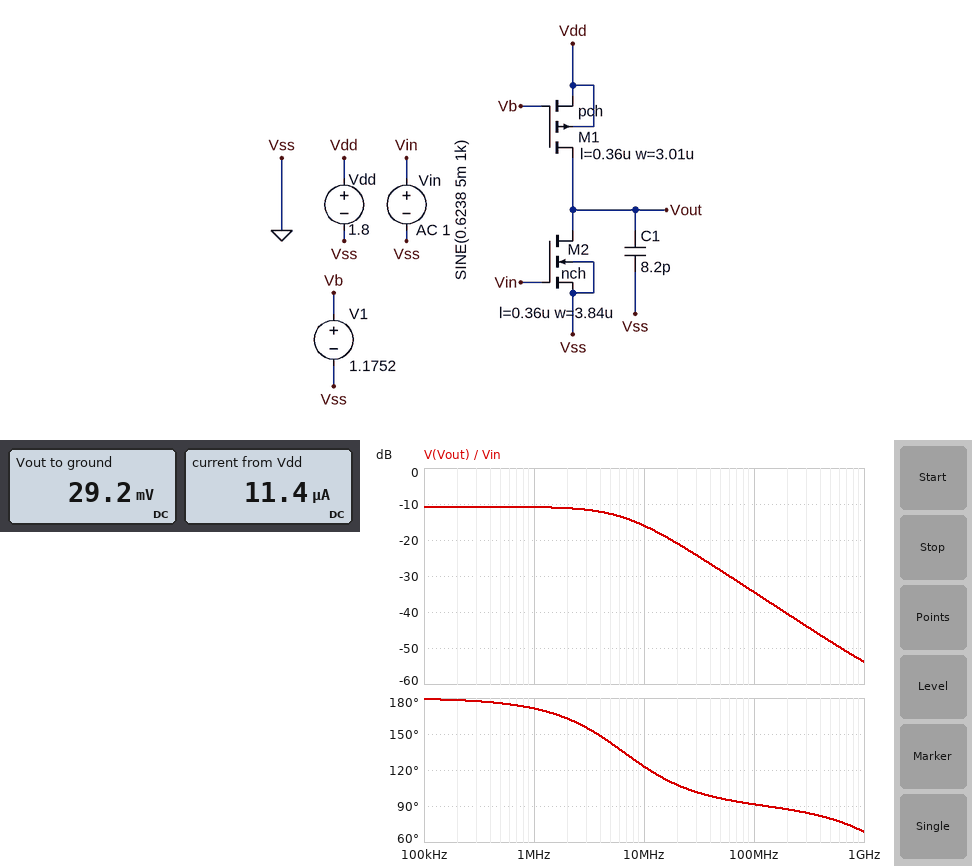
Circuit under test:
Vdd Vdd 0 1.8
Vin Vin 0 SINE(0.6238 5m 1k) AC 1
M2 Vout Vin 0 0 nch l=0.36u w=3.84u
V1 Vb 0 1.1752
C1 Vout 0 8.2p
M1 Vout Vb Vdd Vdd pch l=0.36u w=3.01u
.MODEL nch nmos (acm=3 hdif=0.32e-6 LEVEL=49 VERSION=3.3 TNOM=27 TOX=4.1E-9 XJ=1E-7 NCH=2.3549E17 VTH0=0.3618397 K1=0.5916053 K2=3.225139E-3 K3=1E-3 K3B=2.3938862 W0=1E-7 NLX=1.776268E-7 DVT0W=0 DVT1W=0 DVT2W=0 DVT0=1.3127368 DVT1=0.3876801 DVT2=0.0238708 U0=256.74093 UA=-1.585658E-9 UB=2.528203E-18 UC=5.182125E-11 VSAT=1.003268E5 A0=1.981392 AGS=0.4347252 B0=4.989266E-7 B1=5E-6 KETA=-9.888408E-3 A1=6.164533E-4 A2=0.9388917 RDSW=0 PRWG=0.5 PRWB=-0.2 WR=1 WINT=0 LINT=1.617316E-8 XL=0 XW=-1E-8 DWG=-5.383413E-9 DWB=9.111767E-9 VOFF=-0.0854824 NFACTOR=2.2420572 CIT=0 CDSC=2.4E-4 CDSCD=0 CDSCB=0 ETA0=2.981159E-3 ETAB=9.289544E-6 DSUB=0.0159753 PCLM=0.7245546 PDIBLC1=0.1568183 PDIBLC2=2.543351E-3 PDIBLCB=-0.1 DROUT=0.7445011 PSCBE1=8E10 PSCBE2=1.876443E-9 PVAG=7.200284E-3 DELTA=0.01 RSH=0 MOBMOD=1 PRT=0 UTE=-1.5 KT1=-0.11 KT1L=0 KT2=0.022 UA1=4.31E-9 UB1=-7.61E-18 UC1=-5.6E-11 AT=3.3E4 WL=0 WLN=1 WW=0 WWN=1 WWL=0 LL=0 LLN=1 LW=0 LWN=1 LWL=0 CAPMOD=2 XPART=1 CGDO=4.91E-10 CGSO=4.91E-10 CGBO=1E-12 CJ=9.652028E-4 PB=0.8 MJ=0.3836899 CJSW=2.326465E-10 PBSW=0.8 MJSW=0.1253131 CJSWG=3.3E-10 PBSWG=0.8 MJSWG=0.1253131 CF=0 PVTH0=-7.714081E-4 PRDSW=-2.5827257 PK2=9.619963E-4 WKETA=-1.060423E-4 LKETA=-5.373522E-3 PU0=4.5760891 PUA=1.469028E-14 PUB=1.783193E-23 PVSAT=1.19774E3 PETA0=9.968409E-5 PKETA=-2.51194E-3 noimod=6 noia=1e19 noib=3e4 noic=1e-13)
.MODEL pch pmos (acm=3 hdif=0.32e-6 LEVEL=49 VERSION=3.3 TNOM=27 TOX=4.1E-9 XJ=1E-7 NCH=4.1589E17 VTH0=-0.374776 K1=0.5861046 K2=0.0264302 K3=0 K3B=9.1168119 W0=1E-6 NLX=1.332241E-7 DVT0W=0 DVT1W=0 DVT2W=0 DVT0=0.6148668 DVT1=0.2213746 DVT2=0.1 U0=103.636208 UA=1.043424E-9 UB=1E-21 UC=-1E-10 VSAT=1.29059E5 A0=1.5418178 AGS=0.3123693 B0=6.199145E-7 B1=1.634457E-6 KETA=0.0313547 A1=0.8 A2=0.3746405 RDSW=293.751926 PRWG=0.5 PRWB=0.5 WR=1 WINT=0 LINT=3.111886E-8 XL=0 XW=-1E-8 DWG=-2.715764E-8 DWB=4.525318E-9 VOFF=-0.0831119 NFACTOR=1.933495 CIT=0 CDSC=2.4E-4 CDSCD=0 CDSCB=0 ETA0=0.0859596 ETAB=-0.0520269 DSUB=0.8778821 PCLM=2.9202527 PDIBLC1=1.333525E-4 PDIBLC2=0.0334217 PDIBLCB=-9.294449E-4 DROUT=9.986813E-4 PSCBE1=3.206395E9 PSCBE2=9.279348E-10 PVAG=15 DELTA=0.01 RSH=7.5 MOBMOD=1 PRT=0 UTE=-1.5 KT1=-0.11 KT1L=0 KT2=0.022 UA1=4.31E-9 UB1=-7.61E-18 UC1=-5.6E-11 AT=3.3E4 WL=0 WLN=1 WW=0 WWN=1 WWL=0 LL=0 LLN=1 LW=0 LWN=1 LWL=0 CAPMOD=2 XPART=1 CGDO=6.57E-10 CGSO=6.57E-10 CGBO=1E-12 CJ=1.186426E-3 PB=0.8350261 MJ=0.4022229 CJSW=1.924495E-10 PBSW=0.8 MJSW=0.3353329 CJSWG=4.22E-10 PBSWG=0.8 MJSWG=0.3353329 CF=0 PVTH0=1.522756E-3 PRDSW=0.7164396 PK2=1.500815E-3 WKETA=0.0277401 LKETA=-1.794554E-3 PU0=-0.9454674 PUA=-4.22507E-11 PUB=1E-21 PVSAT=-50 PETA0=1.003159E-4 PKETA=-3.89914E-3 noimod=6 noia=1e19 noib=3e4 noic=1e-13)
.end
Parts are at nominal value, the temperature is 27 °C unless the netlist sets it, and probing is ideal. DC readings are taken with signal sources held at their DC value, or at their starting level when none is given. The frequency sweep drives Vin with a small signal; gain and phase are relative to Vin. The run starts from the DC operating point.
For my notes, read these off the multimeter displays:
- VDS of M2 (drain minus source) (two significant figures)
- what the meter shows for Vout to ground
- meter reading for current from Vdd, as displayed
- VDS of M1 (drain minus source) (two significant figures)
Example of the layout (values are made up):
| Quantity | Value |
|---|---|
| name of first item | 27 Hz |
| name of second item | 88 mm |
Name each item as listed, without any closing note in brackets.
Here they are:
| Quantity | Value |
|---|---|
| VDS of M2 (drain minus source) | 29 mV |
| what the meter shows for Vout to ground | 29.2 mV |
| meter reading for current from Vdd, as displayed | 11.4 µA |
| VDS of M1 (drain minus source) | -1.8 V |
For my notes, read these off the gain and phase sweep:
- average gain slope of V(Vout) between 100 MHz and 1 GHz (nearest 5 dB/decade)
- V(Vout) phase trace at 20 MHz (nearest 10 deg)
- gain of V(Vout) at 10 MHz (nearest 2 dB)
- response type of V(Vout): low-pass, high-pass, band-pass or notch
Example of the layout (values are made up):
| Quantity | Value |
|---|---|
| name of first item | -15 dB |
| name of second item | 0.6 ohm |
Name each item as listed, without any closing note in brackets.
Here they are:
| Quantity | Value |
|---|---|
| average gain slope of V(Vout) between 100 MHz and 1 GHz | -20 dB/decade |
| V(Vout) phase trace at 20 MHz | 110 deg |
| gain of V(Vout) at 10 MHz | -16 dB |
| response type of V(Vout): low-pass, high-pass, band-pass or notch | low-pass |
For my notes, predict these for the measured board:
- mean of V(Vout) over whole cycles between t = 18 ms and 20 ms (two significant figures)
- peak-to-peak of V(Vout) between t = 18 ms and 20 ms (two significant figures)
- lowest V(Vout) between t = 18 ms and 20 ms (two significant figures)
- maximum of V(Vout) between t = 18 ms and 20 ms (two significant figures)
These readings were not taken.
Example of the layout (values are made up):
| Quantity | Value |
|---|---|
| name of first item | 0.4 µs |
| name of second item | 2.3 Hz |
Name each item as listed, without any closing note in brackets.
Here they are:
| Quantity | Value |
|---|---|
| mean of V(Vout) over whole cycles between t = 18 ms and 20 ms | 29 mV |
| peak-to-peak of V(Vout) between t = 18 ms and 20 ms | 2.9 mV |
| lowest V(Vout) between t = 18 ms and 20 ms | 28 mV |
| maximum of V(Vout) between t = 18 ms and 20 ms | 31 mV |
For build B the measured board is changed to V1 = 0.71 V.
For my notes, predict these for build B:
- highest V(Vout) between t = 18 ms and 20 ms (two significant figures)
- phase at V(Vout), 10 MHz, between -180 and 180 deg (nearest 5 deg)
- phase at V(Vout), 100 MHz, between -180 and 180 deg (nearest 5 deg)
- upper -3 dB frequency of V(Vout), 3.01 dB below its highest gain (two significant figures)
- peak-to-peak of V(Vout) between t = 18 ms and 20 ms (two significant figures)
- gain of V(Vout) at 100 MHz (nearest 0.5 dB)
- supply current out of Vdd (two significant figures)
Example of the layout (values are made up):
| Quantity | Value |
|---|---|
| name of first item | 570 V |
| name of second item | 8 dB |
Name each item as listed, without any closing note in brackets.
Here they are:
| Quantity | Value |
|---|---|
| highest V(Vout) between t = 18 ms and 20 ms | 1.7 V |
| phase at V(Vout), 10 MHz, between -180 and 180 deg | 120 deg |
| phase at V(Vout), 100 MHz, between -180 and 180 deg | 95 deg |
| upper -3 dB frequency of V(Vout), 3.01 dB below its highest gain | 5.7 MHz |
| peak-to-peak of V(Vout) between t = 18 ms and 20 ms | 16 mV |
| gain of V(Vout) at 100 MHz | -21.0 dB |
| supply current out of Vdd | 40 µA |
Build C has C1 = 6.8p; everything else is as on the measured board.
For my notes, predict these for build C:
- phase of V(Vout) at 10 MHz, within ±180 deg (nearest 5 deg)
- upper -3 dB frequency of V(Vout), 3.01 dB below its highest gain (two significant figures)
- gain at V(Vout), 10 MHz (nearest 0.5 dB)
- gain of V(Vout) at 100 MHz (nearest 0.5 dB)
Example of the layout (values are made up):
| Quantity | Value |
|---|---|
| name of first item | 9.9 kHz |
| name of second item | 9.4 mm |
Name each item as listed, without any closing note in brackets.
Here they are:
| Quantity | Value |
|---|---|
| phase of V(Vout) at 10 MHz, within ±180 deg | 130 deg |
| upper -3 dB frequency of V(Vout), 3.01 dB below its highest gain | 7.9 MHz |
| gain at V(Vout), 10 MHz | -15.0 dB |
| gain of V(Vout) at 100 MHz | -33.0 dB |
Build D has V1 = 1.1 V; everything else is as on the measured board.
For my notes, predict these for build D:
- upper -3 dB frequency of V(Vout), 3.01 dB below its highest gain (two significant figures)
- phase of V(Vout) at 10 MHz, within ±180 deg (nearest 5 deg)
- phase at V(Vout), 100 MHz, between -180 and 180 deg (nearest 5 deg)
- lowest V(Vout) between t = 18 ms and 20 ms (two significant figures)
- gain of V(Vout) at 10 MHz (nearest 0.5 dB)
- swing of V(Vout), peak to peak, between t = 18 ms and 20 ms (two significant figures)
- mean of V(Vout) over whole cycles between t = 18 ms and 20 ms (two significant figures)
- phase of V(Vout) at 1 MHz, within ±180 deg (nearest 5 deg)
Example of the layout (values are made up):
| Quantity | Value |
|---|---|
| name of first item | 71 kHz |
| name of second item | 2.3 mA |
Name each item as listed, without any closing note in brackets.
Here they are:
| Quantity | Value |
|---|---|
| upper -3 dB frequency of V(Vout), 3.01 dB below its highest gain | 4.0 MHz |
| phase of V(Vout) at 10 MHz, within ±180 deg | 110 deg |
| phase at V(Vout), 100 MHz, between -180 and 180 deg | 90 deg |
| lowest V(Vout) between t = 18 ms and 20 ms | 63 mV |
| gain of V(Vout) at 10 MHz | -8.5 dB |
| swing of V(Vout), peak to peak, between t = 18 ms and 20 ms | 10 mV |
| mean of V(Vout) over whole cycles between t = 18 ms and 20 ms | 68 mV |
| phase of V(Vout) at 1 MHz, within ±180 deg | 165 deg |
